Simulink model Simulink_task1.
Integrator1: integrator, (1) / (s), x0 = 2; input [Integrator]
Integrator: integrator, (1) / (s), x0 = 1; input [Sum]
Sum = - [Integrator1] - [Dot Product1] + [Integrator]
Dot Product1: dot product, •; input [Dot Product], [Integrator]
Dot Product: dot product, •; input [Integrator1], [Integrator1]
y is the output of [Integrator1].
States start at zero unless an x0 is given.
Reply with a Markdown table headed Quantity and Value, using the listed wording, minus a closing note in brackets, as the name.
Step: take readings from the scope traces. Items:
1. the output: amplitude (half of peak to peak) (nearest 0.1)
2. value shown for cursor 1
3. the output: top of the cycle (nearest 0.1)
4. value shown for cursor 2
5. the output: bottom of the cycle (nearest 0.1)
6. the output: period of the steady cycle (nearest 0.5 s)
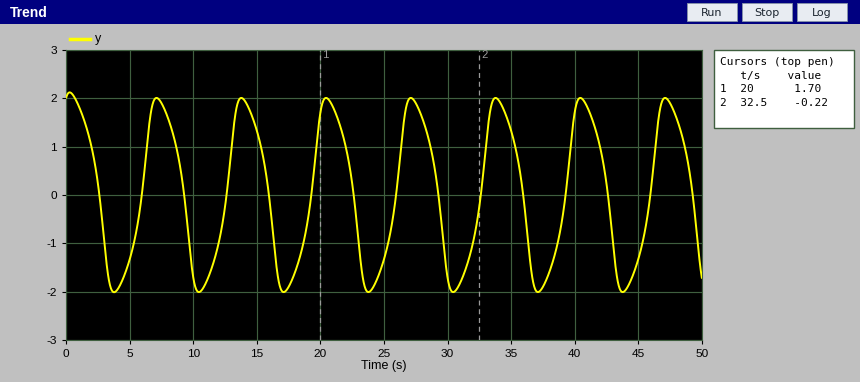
| Quantity | Value |
|---|---|
| the output: amplitude (half of peak to peak) | 2.0 |
| value shown for cursor 1 | 1.70 |
| the output: top of the cycle | 2.0 |
| value shown for cursor 2 | -0.22 |
| the output: bottom of the cycle | -2.0 |
| the output: period of the steady cycle | 6.5 s |
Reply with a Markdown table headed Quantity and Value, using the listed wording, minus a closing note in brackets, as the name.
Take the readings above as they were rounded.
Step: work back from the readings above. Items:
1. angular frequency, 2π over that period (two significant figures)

| Quantity | Value |
|---|---|
| angular frequency, 2π over that period | 0.97 rad/s |
